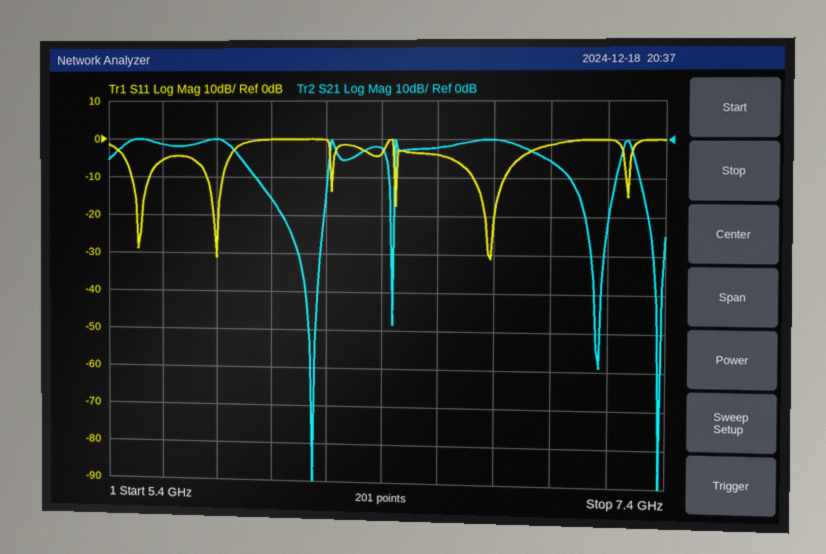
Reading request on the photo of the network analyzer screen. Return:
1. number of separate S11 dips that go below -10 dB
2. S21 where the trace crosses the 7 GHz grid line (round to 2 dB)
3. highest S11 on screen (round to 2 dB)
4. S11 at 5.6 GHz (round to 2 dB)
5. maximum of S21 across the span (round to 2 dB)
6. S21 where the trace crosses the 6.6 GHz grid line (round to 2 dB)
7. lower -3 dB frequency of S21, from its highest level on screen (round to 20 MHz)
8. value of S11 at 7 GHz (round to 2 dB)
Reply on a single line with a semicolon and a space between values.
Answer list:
6; -6 dB; 0 dB; -6 dB; 0 dB; -2 dB; 5.44 GHz; -2 dB
